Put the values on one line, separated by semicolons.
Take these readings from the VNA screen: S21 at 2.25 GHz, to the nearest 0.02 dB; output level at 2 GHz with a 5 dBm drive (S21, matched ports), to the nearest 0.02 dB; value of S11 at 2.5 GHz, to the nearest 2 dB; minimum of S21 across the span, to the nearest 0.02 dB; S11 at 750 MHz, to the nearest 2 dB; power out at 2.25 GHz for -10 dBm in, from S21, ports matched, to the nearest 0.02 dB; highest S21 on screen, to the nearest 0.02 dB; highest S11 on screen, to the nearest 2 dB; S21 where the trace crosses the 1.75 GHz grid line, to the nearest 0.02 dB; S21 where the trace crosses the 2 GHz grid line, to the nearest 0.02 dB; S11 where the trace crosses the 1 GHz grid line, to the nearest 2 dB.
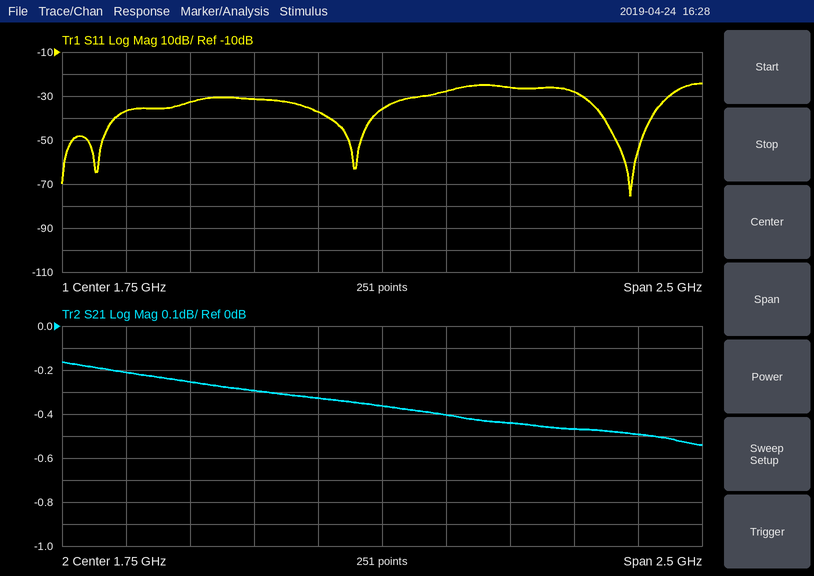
-0.44 dB; 4.60 dBm; -28 dB; -0.54 dB; -36 dB; -10.44 dBm; -0.16 dB; -24 dB; -0.36 dB; -0.40 dB; -32 dB
